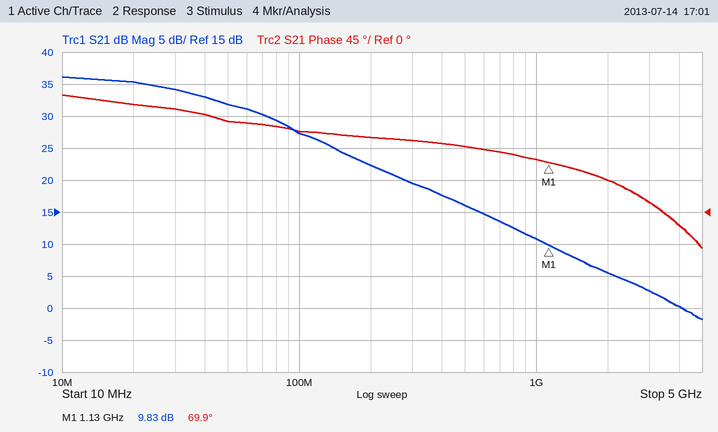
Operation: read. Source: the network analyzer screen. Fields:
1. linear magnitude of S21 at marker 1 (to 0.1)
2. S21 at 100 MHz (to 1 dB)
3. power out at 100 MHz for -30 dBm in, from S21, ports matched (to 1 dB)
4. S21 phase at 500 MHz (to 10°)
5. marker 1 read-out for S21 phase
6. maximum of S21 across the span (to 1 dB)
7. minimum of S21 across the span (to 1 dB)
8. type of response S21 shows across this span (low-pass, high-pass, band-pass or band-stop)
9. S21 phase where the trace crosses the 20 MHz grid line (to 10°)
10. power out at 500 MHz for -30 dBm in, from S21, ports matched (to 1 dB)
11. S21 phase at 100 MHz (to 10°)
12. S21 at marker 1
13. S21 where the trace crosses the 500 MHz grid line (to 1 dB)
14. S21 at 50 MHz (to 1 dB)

3.1
27 dB
-3 dBm
90°
69.9°
36 dB
-2 dB
low-pass
150°
-14 dBm
110°
9.83 dB
16 dB
32 dB
